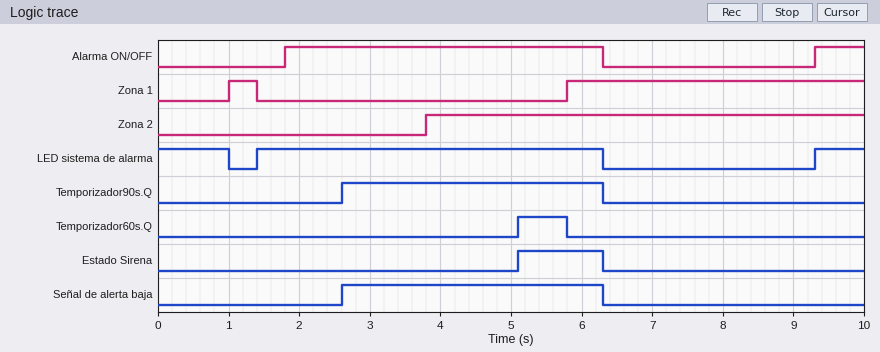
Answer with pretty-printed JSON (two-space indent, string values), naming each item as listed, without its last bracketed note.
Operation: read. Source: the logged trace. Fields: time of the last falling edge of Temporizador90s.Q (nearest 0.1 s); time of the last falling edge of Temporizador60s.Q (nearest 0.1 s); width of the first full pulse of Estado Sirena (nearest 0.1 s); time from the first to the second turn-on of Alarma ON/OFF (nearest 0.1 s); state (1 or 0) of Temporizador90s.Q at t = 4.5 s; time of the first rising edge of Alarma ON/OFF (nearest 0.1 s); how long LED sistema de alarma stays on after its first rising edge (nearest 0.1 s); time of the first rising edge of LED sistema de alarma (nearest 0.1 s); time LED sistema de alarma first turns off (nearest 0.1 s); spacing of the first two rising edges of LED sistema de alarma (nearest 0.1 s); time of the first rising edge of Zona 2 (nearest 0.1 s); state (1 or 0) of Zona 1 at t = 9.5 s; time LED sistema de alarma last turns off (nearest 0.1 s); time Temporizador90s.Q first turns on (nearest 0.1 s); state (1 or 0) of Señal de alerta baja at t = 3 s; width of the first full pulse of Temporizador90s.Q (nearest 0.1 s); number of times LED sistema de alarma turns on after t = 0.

{
  "time of the last falling edge of Temporizador90s.Q": "6.3 s",
  "time of the last falling edge of Temporizador60s.Q": "5.8 s",
  "width of the first full pulse of Estado Sirena": "1.2 s",
  "time from the first to the second turn-on of Alarma ON/OFF": "7.5 s",
  "state (1 or 0) of Temporizador90s.Q at t = 4.5 s": "1",
  "time of the first rising edge of Alarma ON/OFF": "1.8 s",
  "how long LED sistema de alarma stays on after its first rising edge": "4.9 s",
  "time of the first rising edge of LED sistema de alarma": "1.4 s",
  "time LED sistema de alarma first turns off": "1.0 s",
  "spacing of the first two rising edges of LED sistema de alarma": "7.9 s",
  "time of the first rising edge of Zona 2": "3.8 s",
  "state (1 or 0) of Zona 1 at t = 9.5 s": "1",
  "time LED sistema de alarma last turns off": "6.3 s",
  "time Temporizador90s.Q first turns on": "2.6 s",
  "state (1 or 0) of Señal de alerta baja at t = 3 s": "1",
  "width of the first full pulse of Temporizador90s.Q": "3.7 s",
  "number of times LED sistema de alarma turns on after t = 0": "2"
}
